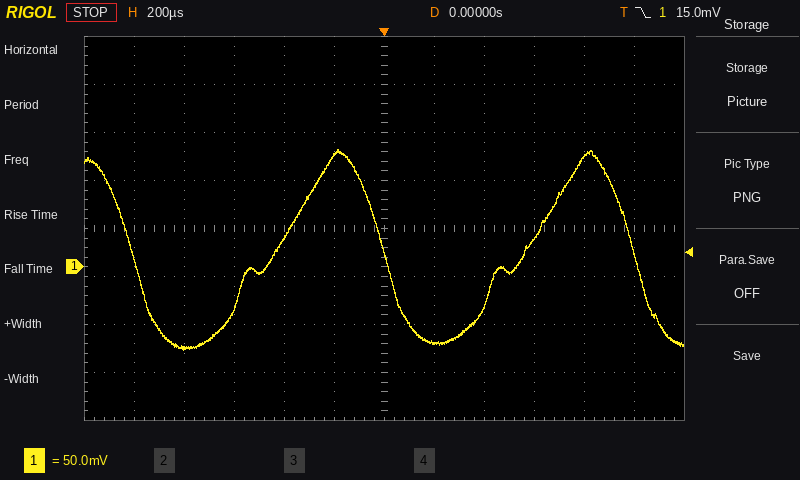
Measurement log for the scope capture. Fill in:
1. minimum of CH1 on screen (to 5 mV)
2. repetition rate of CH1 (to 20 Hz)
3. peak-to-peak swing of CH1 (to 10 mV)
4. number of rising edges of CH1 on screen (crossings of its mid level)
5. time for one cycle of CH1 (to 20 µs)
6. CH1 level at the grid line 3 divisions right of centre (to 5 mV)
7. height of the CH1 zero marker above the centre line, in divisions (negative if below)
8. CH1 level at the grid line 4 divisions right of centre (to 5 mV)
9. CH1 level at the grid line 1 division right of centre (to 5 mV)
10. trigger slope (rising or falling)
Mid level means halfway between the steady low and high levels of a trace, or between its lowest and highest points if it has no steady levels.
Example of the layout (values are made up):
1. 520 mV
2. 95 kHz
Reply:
1. -85 mV
2. 1.00 kHz
3. 210 mV
4. 2
5. 1.00 ms
6. 30 mV
7. -0.8 div
8. 115 mV
9. -80 mV
10. falling
